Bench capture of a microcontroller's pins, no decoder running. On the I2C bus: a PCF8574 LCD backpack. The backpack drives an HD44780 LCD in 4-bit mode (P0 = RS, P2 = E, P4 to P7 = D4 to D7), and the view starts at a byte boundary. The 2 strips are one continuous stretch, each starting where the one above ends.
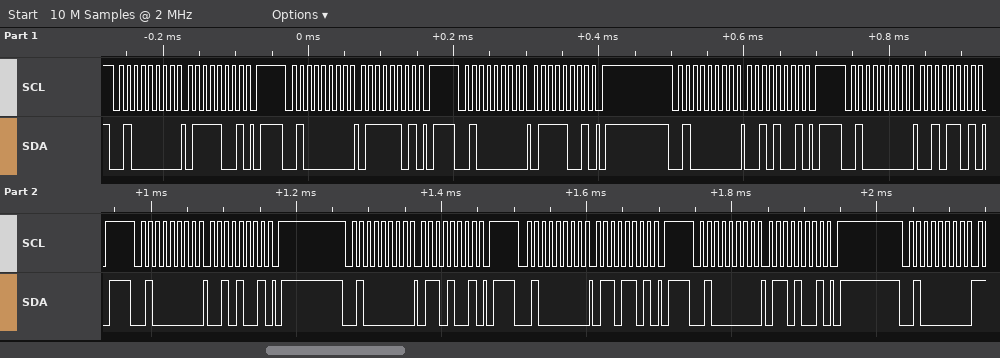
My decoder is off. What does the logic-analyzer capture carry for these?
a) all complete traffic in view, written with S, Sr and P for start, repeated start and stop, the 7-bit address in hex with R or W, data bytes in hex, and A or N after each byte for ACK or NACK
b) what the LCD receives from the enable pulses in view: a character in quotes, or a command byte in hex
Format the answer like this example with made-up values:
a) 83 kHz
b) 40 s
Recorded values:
a) S 20W A 79 A P S 20W A 7D A P S 20W A 79 A P S 20W A 29 A P S 20W A 2D A P S 20W A 29 A P S 20W A 69 A P S 20W A 6D A P S 20W A 69 A P S 20W A
b) 'r'
